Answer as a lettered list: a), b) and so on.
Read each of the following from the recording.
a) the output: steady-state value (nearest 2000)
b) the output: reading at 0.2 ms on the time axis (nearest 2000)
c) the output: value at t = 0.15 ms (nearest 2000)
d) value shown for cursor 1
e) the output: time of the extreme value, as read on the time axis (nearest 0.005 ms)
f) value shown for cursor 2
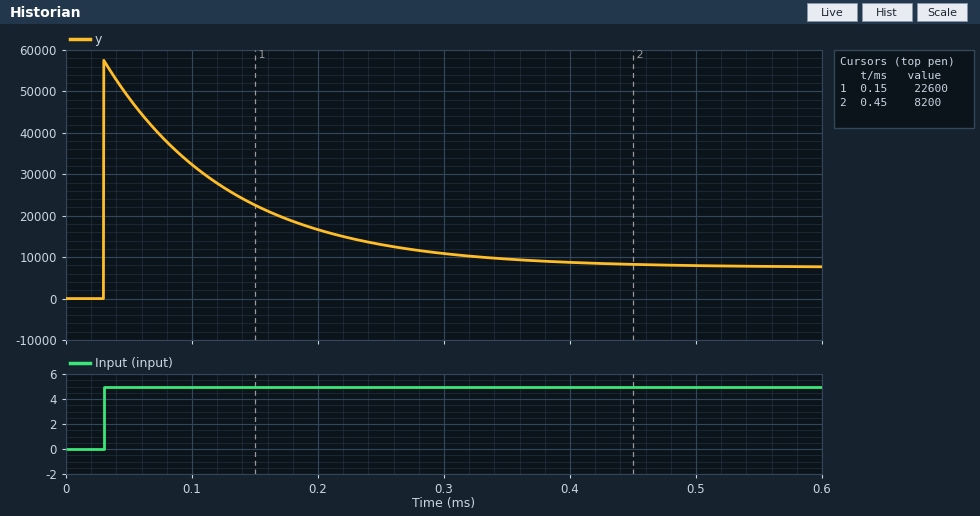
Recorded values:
a) 8000
b) 16000
c) 22000
d) 22600
e) 0.030 ms
f) 8200
